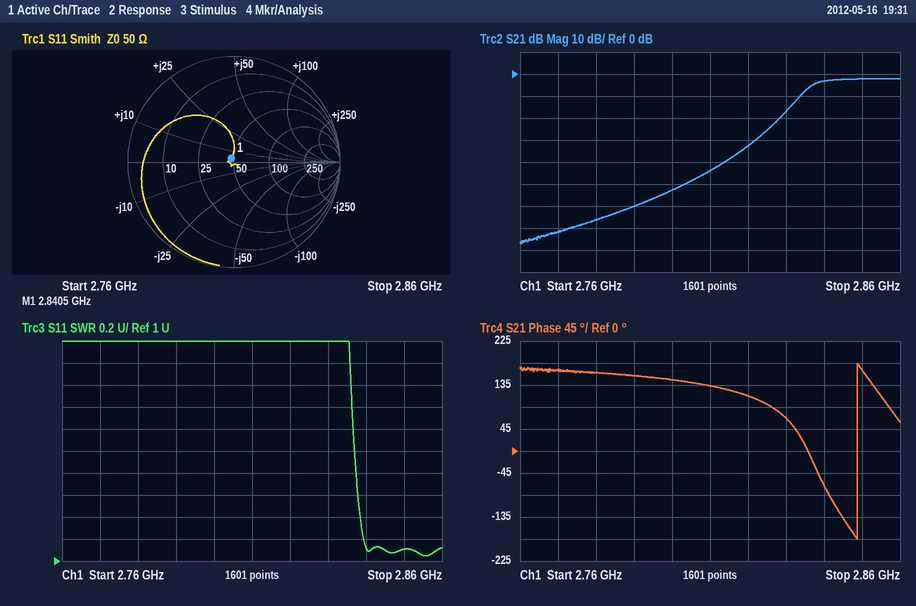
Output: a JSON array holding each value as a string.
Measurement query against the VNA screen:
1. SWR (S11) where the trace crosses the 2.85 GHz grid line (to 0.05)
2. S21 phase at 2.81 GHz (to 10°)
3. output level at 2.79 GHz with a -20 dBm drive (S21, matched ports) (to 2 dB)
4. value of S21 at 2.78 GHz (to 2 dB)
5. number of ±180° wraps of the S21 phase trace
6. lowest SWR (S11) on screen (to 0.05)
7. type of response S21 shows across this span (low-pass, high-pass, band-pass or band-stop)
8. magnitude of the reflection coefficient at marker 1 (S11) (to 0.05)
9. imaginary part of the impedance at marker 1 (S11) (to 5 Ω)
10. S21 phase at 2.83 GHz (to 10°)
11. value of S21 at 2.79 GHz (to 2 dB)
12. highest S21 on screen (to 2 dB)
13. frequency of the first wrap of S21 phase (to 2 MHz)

["1.10", "130°", "-80 dBm", "-66 dB", "1", "1.05", "high-pass", "0.05", "+5 Ω", "70°", "-60 dB", "-2 dB", "2.848 GHz"]
